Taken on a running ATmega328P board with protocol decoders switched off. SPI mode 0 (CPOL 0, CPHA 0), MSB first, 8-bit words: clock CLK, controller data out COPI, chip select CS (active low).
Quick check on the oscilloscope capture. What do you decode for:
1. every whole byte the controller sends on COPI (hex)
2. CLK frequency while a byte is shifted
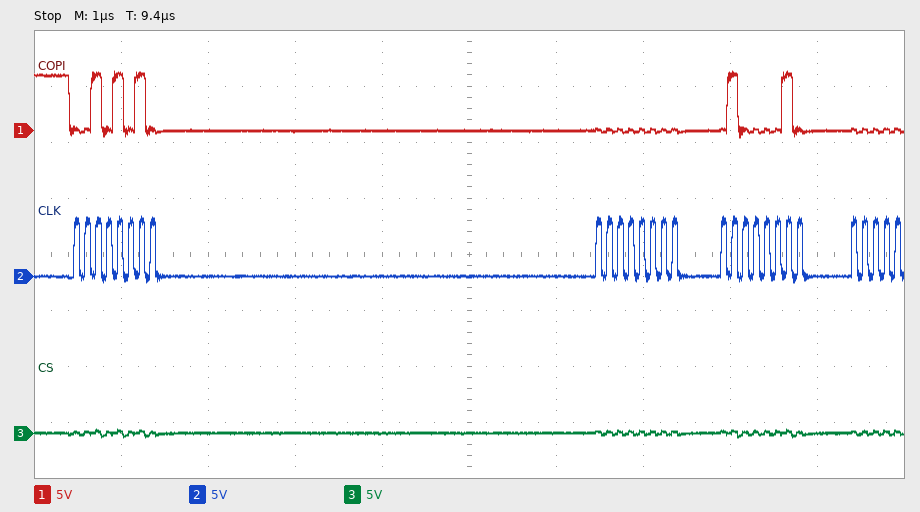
2A 00 42
8 MHz
